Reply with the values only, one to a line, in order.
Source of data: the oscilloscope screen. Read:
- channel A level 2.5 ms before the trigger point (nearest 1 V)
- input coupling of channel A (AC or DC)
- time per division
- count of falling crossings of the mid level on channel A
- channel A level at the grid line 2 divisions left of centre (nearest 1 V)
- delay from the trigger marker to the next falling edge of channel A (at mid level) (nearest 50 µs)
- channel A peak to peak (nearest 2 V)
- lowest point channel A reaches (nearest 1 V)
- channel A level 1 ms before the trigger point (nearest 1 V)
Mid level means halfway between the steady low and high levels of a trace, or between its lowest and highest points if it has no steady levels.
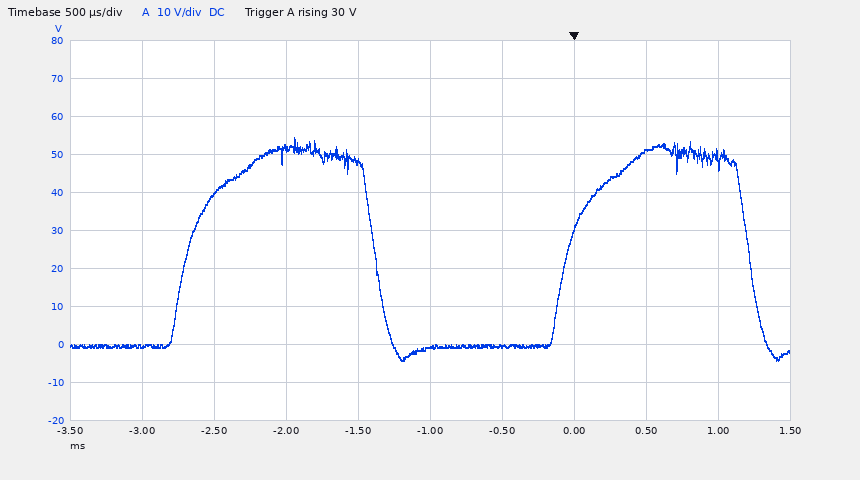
40 V
DC
500 µs
2
52 V
1.20 ms
58 V
-4 V
-1 V
